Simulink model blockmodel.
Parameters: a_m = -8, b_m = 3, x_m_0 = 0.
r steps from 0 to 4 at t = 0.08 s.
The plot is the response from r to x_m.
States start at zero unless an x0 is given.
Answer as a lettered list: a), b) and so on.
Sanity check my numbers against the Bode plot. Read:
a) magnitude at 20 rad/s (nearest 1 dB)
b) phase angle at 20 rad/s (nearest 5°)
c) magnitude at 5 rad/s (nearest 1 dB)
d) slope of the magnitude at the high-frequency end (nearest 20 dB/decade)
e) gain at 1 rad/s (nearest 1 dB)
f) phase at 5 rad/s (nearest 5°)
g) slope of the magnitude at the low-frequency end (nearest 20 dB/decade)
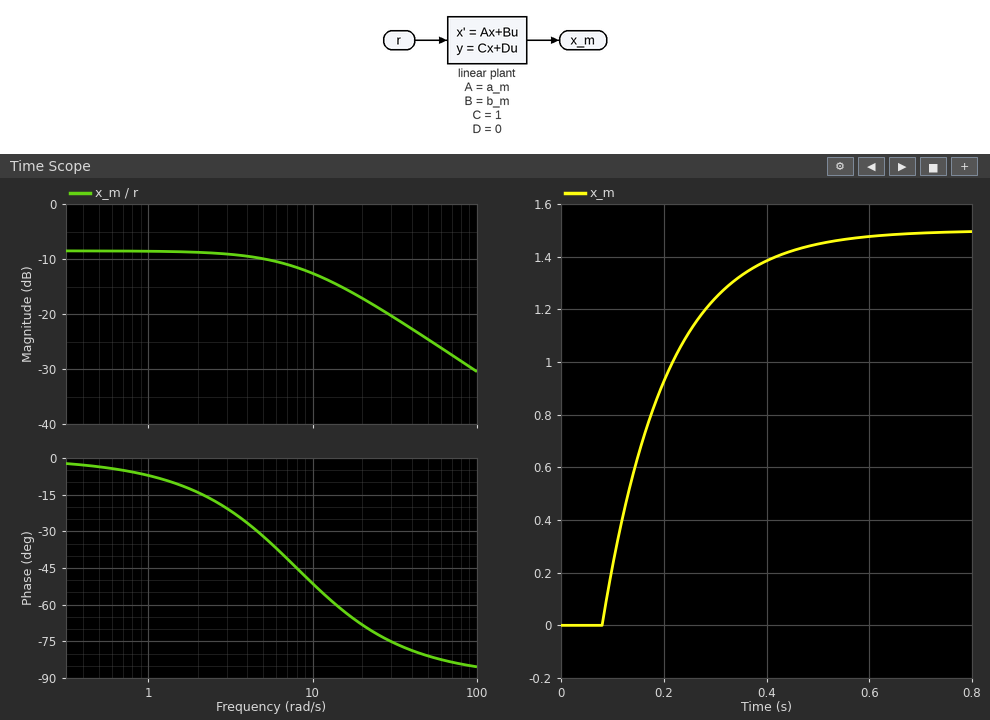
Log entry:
a) -17 dB
b) -70°
c) -10 dB
d) -20 dB/decade
e) -9 dB
f) -30°
g) 0 dB/decade
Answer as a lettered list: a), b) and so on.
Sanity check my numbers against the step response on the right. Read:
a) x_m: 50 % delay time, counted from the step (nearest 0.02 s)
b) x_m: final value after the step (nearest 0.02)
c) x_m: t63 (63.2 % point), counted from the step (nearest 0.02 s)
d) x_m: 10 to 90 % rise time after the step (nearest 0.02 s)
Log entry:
a) 0.08 s
b) 1.50
c) 0.12 s
d) 0.28 s
